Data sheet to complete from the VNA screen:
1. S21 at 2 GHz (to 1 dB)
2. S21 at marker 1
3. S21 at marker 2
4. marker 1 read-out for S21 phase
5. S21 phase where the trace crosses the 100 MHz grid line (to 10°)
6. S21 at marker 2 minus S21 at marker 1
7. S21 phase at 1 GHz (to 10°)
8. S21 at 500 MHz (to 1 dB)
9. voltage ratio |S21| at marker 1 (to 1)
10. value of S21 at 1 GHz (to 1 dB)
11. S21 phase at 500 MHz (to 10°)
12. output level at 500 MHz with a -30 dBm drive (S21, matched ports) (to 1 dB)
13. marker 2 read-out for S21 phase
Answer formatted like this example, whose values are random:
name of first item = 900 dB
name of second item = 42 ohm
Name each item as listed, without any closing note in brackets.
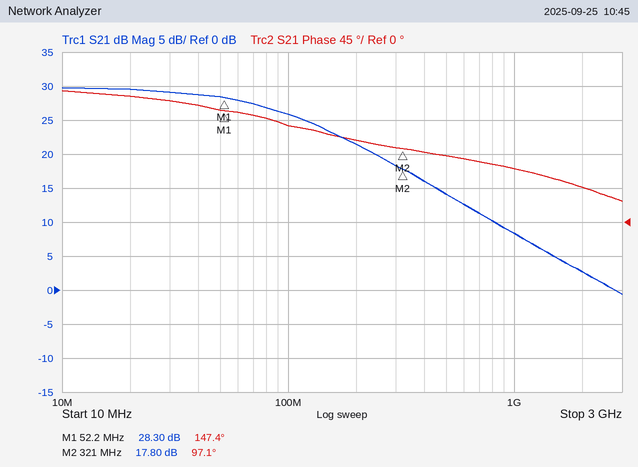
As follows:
S21 at 2 GHz = 3 dB
S21 at marker 1 = 28.30 dB
S21 at marker 2 = 17.80 dB
marker 1 read-out for S21 phase = 147.4°
S21 phase where the trace crosses the 100 MHz grid line = 130°
S21 at marker 2 minus S21 at marker 1 = -10.50 dB
S21 phase at 1 GHz = 70°
S21 at 500 MHz = 14 dB
voltage ratio |S21| at marker 1 = 26
value of S21 at 1 GHz = 8 dB
S21 phase at 500 MHz = 90°
output level at 500 MHz with a -30 dBm drive (S21, matched ports) = -16 dBm
marker 2 read-out for S21 phase = 97.1°
